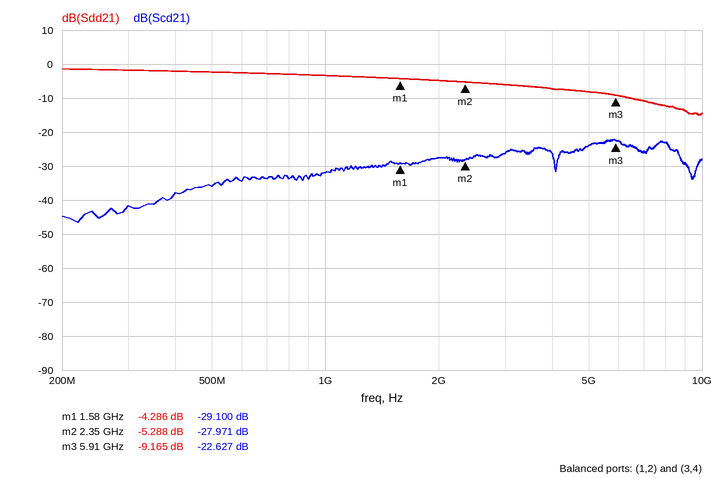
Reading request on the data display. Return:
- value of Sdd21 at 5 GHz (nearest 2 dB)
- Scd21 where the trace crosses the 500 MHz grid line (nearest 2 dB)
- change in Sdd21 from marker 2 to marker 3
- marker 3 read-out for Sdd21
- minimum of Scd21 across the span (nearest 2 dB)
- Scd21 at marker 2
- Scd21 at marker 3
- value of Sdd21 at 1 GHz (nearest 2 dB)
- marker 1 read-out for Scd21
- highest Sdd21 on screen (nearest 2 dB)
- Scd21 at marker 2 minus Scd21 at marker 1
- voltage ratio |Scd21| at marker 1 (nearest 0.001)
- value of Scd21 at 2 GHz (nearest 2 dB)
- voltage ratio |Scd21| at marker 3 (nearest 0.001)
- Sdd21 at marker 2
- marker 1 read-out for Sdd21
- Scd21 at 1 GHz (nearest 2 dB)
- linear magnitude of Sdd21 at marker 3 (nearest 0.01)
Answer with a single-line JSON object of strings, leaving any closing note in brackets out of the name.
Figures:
{"value of Sdd21 at 5 GHz": "-8 dB", "Scd21 where the trace crosses the 500 MHz grid line": "-36 dB", "change in Sdd21 from marker 2 to marker 3": "-3.877 dB", "marker 3 read-out for Sdd21": "-9.165 dB", "minimum of Scd21 across the span": "-46 dB", "Scd21 at marker 2": "-27.971 dB", "Scd21 at marker 3": "-22.627 dB", "value of Sdd21 at 1 GHz": "-4 dB", "marker 1 read-out for Scd21": "-29.100 dB", "highest Sdd21 on screen": "-2 dB", "Scd21 at marker 2 minus Scd21 at marker 1": "1.129 dB", "voltage ratio |Scd21| at marker 1": "0.035", "value of Scd21 at 2 GHz": "-28 dB", "voltage ratio |Scd21| at marker 3": "0.074", "Sdd21 at marker 2": "-5.288 dB", "marker 1 read-out for Sdd21": "-4.286 dB", "Scd21 at 1 GHz": "-32 dB", "linear magnitude of Sdd21 at marker 3": "0.35"}
